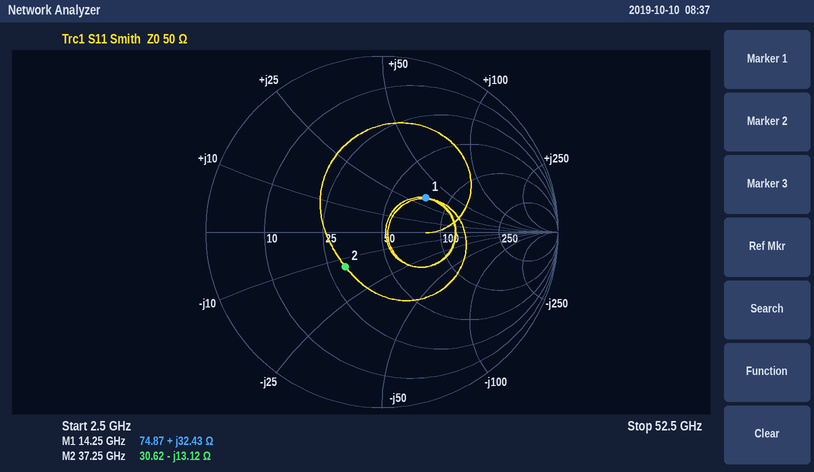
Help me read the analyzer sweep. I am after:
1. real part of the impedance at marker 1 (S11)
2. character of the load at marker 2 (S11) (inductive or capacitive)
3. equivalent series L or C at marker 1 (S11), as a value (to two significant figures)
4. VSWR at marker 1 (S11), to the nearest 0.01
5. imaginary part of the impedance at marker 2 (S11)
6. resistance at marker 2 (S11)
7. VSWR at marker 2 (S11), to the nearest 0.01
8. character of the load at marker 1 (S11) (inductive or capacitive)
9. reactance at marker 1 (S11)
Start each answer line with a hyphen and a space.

- 74.87 Ω
- capacitive
- 360 pH
- 1.93
- -13.12 Ω
- 30.62 Ω
- 1.80
- inductive
- +32.43 Ω
